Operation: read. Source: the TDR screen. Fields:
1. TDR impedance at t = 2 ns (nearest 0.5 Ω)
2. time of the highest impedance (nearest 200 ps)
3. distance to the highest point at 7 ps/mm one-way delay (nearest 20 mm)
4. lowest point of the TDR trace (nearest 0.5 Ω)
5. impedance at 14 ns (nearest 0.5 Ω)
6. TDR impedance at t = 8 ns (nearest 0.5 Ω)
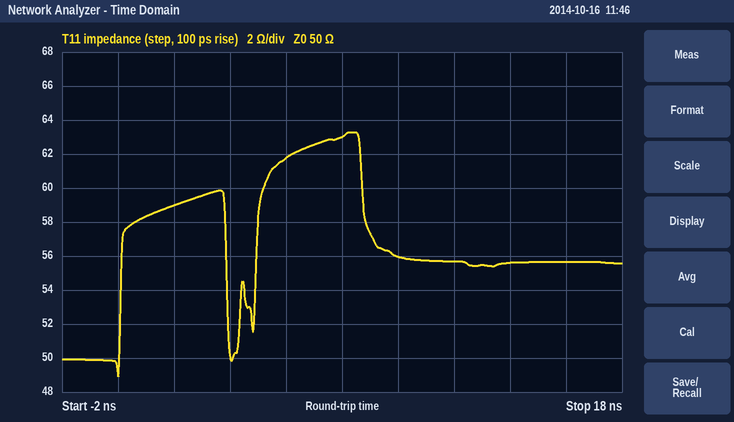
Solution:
59.0 Ω
8.4 ns
600 mm
49.0 Ω
55.5 Ω
63.0 Ω
